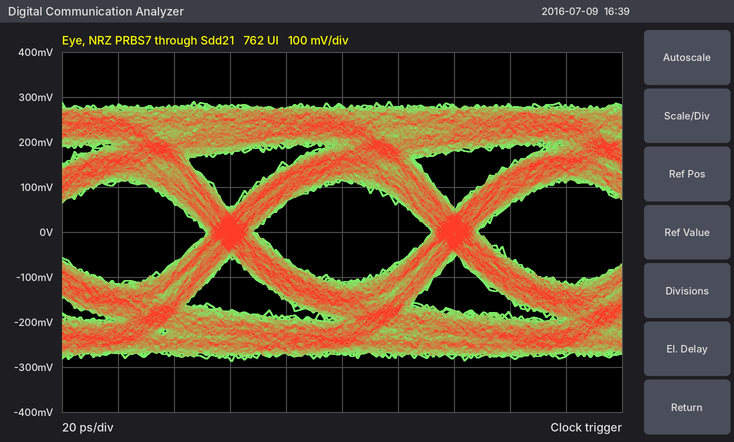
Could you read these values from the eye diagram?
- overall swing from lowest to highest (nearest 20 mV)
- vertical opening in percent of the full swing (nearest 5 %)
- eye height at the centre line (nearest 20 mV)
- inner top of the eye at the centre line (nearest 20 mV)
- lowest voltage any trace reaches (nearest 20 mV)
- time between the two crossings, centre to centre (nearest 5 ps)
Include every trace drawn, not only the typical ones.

580 mV
40 %
220 mV
120 mV
-280 mV
80 ps
